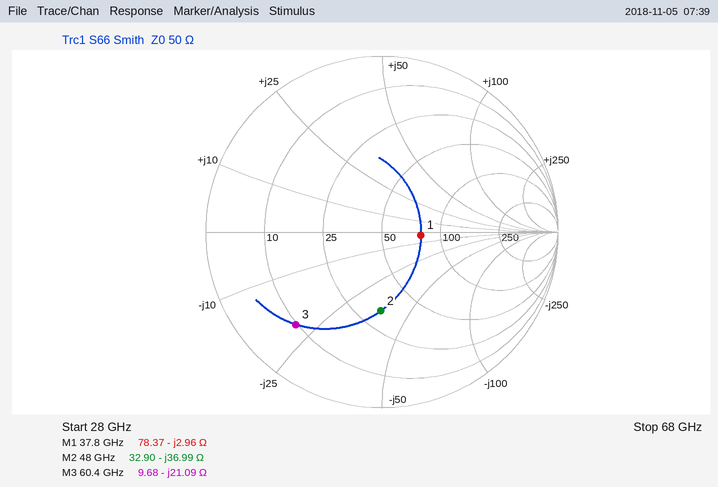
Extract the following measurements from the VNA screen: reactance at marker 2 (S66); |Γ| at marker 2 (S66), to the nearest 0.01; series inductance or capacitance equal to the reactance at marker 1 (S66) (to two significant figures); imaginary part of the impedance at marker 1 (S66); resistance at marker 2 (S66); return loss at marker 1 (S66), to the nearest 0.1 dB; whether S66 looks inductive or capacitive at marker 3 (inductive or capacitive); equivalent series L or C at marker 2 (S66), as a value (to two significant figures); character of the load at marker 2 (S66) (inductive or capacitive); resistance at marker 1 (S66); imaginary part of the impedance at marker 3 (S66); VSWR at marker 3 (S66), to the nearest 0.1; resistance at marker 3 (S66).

-36.99 Ω
0.45
1.4 pF
-2.96 Ω
32.90 Ω
13.1 dB
capacitive
90 fF
capacitive
78.37 Ω
-21.09 Ω
6.1
9.68 Ω
